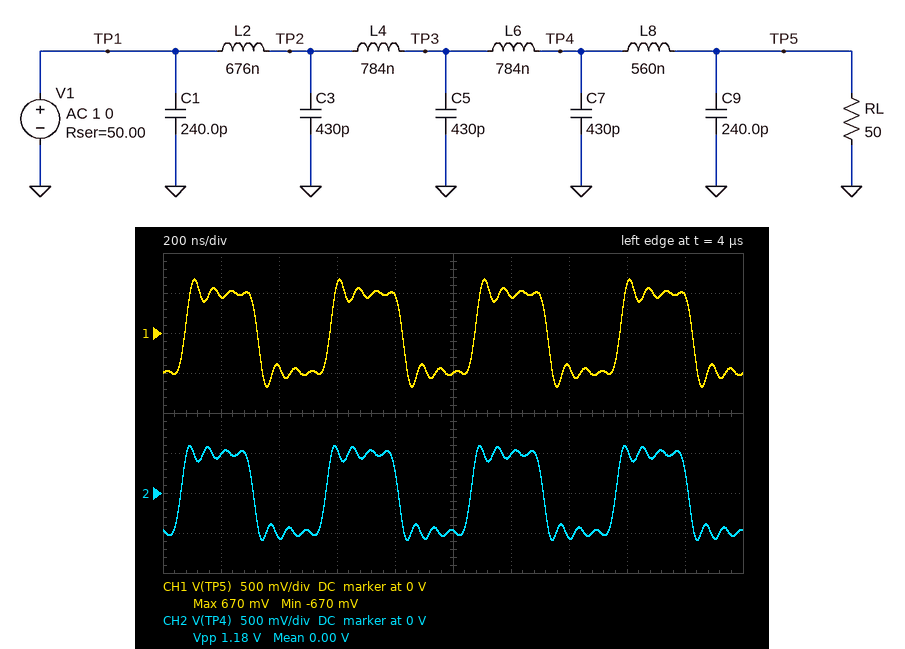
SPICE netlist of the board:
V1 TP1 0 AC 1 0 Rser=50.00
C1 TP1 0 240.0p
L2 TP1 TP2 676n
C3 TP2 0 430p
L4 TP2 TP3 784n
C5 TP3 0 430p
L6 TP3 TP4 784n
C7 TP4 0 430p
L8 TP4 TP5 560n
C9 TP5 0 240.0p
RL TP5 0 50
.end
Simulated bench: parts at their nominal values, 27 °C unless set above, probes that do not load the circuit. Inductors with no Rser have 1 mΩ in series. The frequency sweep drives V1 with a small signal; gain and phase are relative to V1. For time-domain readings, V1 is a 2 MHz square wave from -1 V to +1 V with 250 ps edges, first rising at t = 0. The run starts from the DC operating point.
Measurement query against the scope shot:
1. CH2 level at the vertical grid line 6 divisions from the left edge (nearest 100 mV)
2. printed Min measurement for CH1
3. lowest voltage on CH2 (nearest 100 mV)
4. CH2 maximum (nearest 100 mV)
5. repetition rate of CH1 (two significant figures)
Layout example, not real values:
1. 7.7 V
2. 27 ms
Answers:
1. 500 mV
2. -670 mV
3. -600 mV
4. 600 mV
5. 2.0 MHz
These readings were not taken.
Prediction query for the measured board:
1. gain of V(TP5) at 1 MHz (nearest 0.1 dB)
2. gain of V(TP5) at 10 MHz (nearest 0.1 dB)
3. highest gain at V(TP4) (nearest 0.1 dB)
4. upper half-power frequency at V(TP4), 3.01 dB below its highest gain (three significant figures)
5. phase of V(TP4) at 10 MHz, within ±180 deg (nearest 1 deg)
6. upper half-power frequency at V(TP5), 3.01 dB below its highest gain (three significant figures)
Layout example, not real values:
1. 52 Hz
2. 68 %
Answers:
1. -6.1 dB
2. -6.3 dB
3. -5.0 dB
4. 17.3 MHz
5. 149 deg
6. 17.0 MHz
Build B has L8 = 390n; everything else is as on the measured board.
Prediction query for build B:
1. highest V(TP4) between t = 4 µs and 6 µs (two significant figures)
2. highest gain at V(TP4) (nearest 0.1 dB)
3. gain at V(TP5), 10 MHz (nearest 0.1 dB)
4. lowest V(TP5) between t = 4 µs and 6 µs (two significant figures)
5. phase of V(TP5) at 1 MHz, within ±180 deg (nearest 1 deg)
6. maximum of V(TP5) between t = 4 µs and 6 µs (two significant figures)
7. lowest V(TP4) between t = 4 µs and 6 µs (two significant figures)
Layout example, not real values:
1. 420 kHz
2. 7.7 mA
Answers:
1. 550 mV
2. -6.0 dB
3. -6.7 dB
4. -650 mV
5. -25 deg
6. 650 mV
7. -550 mV
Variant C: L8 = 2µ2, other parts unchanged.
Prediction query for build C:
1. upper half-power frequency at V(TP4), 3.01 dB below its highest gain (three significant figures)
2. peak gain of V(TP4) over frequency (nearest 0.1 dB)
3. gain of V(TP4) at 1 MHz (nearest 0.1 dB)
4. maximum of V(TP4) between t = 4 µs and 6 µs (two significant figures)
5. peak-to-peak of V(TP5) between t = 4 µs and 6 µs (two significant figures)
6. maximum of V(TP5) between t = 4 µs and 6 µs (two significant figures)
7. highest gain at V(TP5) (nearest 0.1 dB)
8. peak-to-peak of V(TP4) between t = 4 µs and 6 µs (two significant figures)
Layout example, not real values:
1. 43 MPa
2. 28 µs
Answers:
1. 16.3 MHz
2. -0.6 dB
3. -5.9 dB
4. 1.0 V
5. 1.1 V
6. 550 mV
7. -6.0 dB
8. 2.1 V
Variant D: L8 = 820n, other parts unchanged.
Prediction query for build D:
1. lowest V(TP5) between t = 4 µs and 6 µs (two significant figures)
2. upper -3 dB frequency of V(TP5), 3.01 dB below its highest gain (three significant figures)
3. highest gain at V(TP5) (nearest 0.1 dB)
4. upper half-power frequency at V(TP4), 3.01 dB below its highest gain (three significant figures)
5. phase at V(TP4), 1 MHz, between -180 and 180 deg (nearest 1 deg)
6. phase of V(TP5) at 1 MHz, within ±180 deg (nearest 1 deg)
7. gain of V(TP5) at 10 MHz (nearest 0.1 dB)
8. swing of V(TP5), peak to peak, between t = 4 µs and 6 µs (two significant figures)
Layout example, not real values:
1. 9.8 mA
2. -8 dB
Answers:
1. -680 mV
2. 16.7 MHz
3. -6.0 dB
4. 16.8 MHz
5. -21 deg
6. -27 deg
7. -6.0 dB
8. 1.4 V
